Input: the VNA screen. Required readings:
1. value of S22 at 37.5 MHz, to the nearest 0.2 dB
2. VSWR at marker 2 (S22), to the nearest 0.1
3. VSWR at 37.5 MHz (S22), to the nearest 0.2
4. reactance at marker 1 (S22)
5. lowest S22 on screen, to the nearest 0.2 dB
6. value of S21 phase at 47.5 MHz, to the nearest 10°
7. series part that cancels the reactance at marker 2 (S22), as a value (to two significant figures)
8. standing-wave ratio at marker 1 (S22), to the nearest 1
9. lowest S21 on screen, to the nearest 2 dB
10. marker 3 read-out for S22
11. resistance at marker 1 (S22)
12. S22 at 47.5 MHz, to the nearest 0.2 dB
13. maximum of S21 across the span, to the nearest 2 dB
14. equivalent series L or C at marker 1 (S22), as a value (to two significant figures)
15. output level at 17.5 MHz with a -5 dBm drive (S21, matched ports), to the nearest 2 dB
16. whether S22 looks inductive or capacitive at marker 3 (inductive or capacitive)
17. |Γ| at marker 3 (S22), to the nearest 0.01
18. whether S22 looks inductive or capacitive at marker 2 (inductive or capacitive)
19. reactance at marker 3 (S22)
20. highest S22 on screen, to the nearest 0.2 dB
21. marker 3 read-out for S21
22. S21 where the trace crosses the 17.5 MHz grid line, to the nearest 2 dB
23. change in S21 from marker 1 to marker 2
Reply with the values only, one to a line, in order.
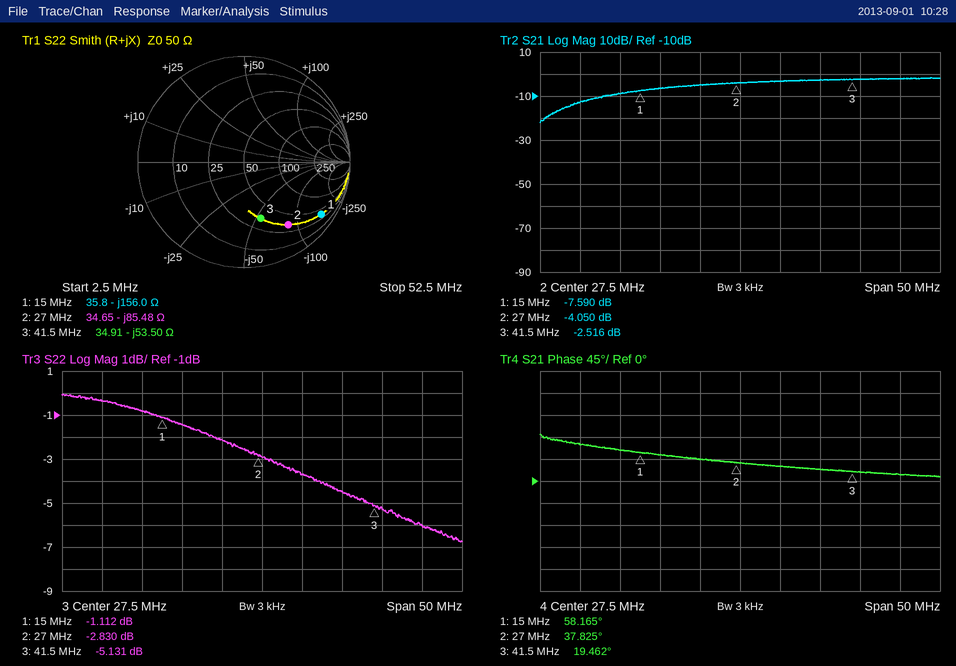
-4.4 dB
6.2
4.0
-156.0 Ω
-6.8 dB
10°
500 nH
16
-22 dB
-5.131 dB
35.8 Ω
-6.0 dB
-2 dB
68 pF
-12 dBm
capacitive
0.55
capacitive
-53.50 Ω
0.0 dB
-2.516 dB
-6 dB
3.540 dB
